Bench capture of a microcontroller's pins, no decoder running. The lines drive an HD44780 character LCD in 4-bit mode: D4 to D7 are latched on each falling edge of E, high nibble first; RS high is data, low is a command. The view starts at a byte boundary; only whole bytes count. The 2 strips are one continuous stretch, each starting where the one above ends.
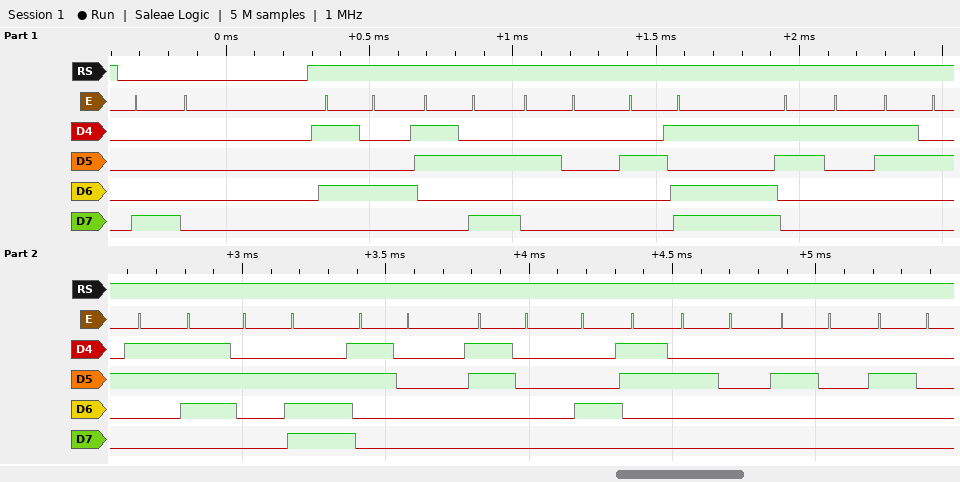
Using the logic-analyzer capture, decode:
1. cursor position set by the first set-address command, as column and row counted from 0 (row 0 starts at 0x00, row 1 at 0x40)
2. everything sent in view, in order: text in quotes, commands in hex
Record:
column 0, row 0
0x80 "T: -127.00C   "
